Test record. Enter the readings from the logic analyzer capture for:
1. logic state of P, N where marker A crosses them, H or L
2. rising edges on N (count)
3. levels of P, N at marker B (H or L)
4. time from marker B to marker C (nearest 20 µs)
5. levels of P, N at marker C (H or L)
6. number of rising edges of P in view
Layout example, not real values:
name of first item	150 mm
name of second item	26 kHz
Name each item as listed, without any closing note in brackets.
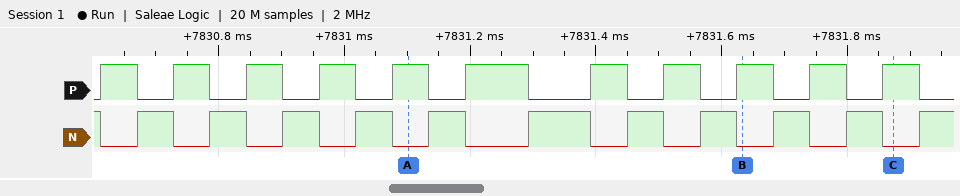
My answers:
logic state of P, N where marker A crosses them, H or L	P=H, N=L
rising edges on N	11
levels of P, N at marker B	P=H, N=L
time from marker B to marker C	240 µs
levels of P, N at marker C	P=H, N=L
number of rising edges of P in view	11
